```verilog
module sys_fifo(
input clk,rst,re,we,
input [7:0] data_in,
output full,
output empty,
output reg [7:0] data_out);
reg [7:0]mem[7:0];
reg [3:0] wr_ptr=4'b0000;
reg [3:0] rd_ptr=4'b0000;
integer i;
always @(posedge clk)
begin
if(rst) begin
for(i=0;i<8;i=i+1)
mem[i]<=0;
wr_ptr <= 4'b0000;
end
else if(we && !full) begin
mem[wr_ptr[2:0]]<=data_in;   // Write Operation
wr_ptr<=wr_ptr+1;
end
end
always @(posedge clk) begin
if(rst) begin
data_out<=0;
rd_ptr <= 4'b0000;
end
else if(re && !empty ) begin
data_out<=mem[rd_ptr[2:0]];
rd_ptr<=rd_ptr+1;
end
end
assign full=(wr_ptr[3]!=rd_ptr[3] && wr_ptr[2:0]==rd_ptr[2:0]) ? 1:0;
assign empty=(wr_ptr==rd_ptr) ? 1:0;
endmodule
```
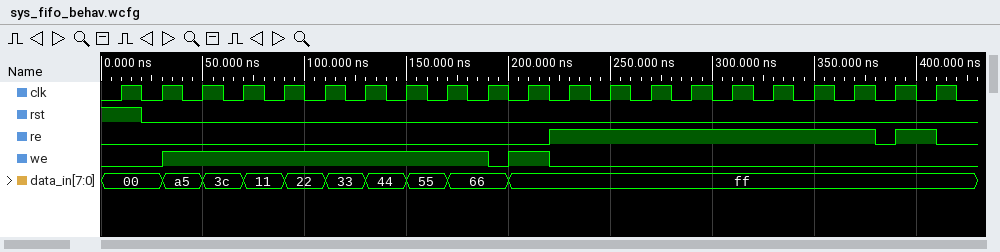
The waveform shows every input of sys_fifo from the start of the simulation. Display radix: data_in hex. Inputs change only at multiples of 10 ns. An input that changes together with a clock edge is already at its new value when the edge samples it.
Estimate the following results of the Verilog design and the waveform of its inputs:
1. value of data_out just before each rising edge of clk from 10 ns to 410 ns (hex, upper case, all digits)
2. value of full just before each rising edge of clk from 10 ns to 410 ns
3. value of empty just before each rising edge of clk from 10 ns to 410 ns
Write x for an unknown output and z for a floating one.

x, 00, 00, 00, 00, 00, 00, 00, 00, 00, 00, 00, A5, 3C, 11, 22, 33, 44, 55, 66, 66
0 0 0 0 0 0 0 0 0 1 1 1 0 0 0 0 0 0 0 0 0
1 1 0 0 0 0 0 0 0 0 0 0 0 0 0 0 0 0 0 1 1
